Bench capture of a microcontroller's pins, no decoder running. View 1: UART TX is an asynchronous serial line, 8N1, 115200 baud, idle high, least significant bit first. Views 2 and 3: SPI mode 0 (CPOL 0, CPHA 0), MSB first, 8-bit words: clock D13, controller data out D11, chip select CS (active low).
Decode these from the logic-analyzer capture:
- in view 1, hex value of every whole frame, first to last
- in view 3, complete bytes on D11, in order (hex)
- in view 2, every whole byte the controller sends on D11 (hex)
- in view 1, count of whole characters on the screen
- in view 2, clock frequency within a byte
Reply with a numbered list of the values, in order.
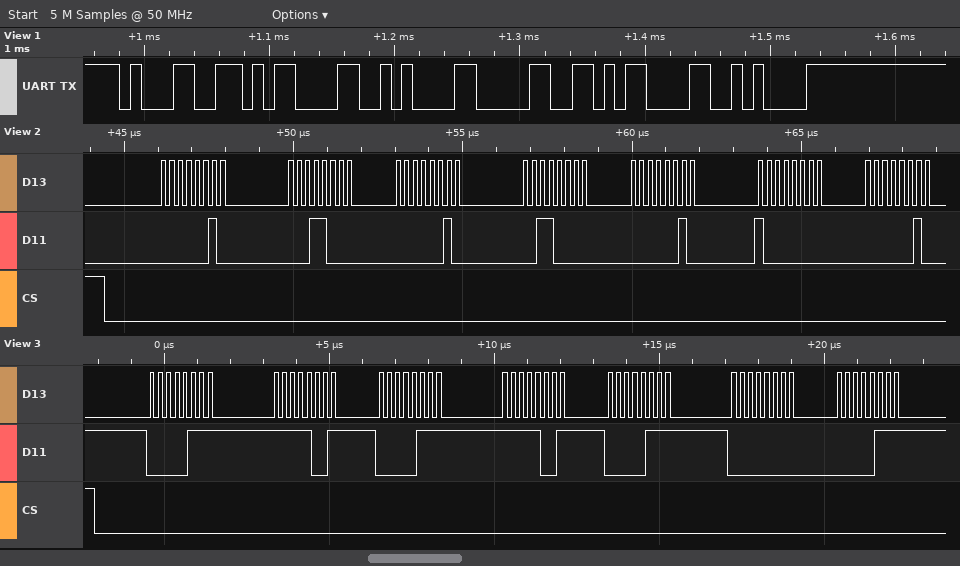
1. 31 0D 0A 30 0D 0A
2. 07 F9 07 F9 07 00 07
3. 02 18 02 30 02 80 02
4. 6
5. 4 MHz
